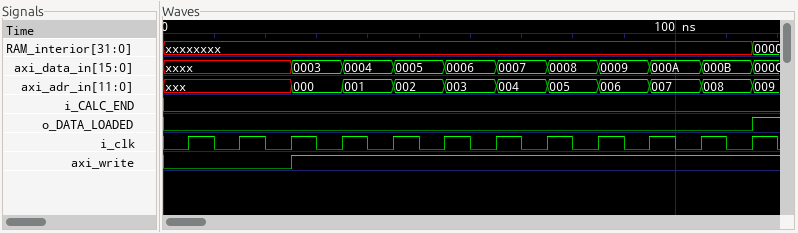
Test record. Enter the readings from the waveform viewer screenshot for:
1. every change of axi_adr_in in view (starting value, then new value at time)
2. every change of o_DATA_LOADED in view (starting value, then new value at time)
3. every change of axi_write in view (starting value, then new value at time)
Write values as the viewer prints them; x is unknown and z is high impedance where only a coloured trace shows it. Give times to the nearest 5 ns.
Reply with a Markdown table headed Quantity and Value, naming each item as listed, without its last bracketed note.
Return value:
| Quantity | Value |
|---|---|
| every change of axi_adr_in in view | xxx, 000 at 25 ns, 001 at 35 ns, 002 at 45 ns, 003 at 55 ns, 004 at 65 ns, 005 at 75 ns, 006 at 85 ns, 007 at 95 ns, 008 at 105 ns, 009 at 115 ns |
| every change of o_DATA_LOADED in view | 0, 1 at 115 ns |
| every change of axi_write in view | 0, 1 at 25 ns |
